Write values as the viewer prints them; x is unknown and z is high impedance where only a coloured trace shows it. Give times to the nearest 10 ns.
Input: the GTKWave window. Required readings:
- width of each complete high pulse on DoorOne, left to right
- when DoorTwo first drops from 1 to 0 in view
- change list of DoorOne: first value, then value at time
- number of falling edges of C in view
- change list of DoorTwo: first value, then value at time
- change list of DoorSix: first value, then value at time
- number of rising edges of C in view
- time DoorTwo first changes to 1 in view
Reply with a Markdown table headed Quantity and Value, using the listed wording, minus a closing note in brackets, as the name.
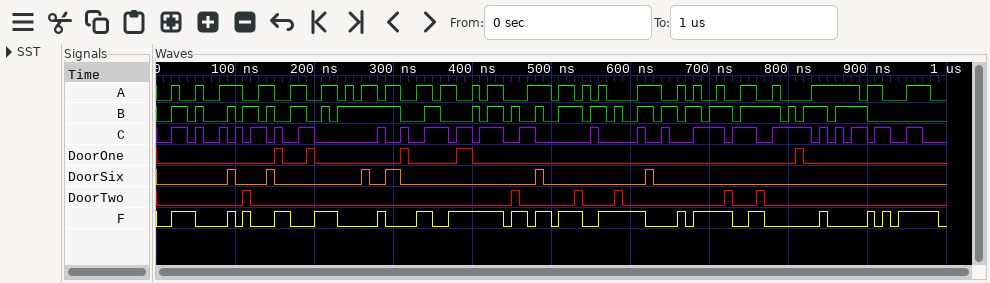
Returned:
| Quantity | Value |
|---|---|
| width of each complete high pulse on DoorOne, left to right | 10 ns, 10 ns, 10 ns, 20 ns, 10 ns |
| when DoorTwo first drops from 1 to 0 in view | 120 ns |
| change list of DoorOne: first value, then value at time | 0, 1 at 150 ns, 0 at 160 ns, 1 at 190 ns, 0 at 200 ns, 1 at 310 ns, 0 at 320 ns, 1 at 380 ns, 0 at 400 ns, 1 at 810 ns, 0 at 820 ns |
| number of falling edges of C in view | 24 |
| change list of DoorTwo: first value, then value at time | 0, 1 at 110 ns, 0 at 120 ns, 1 at 450 ns, 0 at 460 ns, 1 at 530 ns, 0 at 540 ns, 1 at 580 ns, 0 at 590 ns, 1 at 720 ns, 0 at 730 ns, 1 at 760 ns, 0 at 770 ns |
| change list of DoorSix: first value, then value at time | 0, 1 at 90 ns, 0 at 100 ns, 1 at 140 ns, 0 at 150 ns, 1 at 260 ns, 0 at 270 ns, 1 at 290 ns, 0 at 310 ns, 1 at 480 ns, 0 at 490 ns, 1 at 620 ns, 0 at 630 ns |
| number of rising edges of C in view | 24 |
| time DoorTwo first changes to 1 in view | 110 ns |
